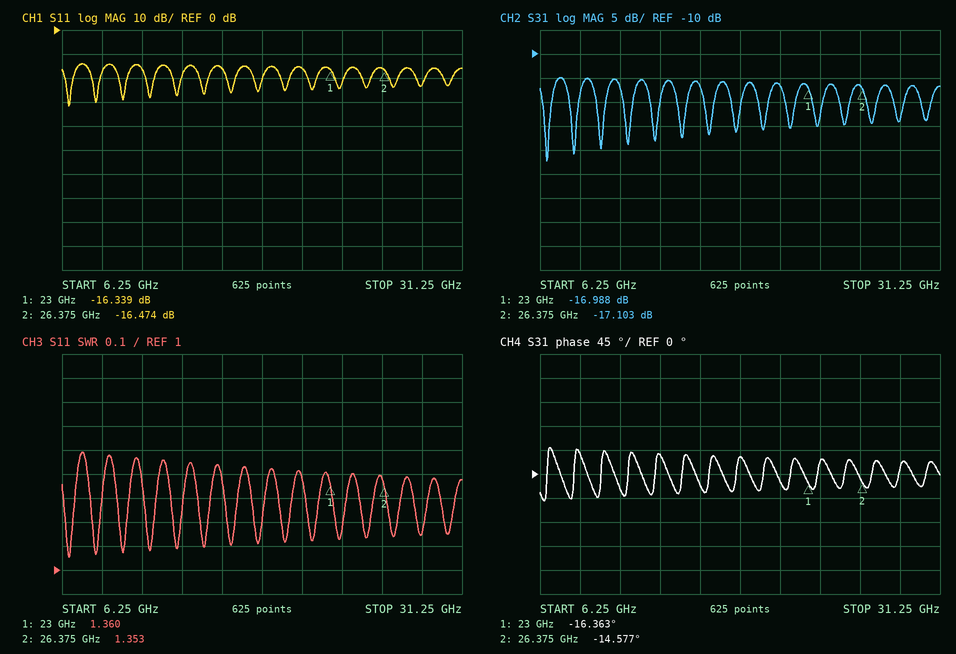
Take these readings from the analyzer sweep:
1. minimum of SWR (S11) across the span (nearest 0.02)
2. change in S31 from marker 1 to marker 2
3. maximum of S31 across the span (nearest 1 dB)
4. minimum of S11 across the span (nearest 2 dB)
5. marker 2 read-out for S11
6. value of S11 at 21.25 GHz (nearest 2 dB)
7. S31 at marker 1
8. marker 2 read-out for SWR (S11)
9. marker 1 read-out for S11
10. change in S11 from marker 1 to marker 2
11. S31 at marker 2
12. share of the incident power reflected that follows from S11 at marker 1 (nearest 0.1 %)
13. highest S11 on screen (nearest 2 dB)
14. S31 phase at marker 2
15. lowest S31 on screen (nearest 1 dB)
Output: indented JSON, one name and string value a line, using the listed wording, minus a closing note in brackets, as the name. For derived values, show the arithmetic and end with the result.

{
  "minimum of SWR (S11) across the span": "1.06",
  "change in S31 from marker 1 to marker 2": "-17.103 − (-16.988) = -0.115 dB",
  "maximum of S31 across the span": "-15 dB",
  "minimum of S11 across the span": "-32 dB",
  "marker 2 read-out for S11": "-16.474 dB",
  "value of S11 at 21.25 GHz": "-16 dB",
  "S31 at marker 1": "-16.988 dB",
  "marker 2 read-out for SWR": "1.353",
  "marker 1 read-out for S11": "-16.339 dB",
  "change in S11 from marker 1 to marker 2": "-16.474 − (-16.339) = -0.135 dB",
  "S31 at marker 2": "-17.103 dB",
  "share of the incident power reflected that follows from S11 at marker 1": "10^(-16.339/10) ≈ 2.3 %",
  "highest S11 on screen": "-14 dB",
  "S31 phase at marker 2": "-14.577°",
  "lowest S31 on screen": "-32 dB"
}
